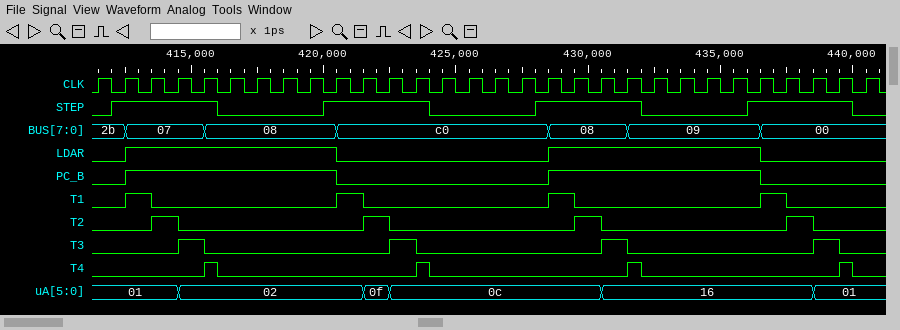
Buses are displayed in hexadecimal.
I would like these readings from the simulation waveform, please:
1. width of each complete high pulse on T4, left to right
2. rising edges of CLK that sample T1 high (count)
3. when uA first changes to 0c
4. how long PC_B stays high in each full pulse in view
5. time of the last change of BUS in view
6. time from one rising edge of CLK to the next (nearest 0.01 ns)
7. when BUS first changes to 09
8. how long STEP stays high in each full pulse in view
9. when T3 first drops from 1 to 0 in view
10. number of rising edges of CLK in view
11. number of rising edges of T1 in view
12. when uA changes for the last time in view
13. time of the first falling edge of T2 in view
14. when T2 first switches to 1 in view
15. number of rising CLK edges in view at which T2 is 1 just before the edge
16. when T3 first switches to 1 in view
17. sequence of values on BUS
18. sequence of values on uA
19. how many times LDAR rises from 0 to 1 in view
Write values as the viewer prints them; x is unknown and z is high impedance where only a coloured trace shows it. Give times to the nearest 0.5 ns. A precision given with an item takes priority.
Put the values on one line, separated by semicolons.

0.5 ns, 0.5 ns, 0.5 ns, 0.5 ns; 4; 422.5 ns; 8 ns, 8 ns; 436.5 ns; 1 ns; 431.5 ns; 4 ns, 4 ns, 4 ns, 4 ns; 415.5 ns; 30; 4; 438.5 ns; 414.5 ns; 413.5 ns; 4; 414.5 ns; 2b, 07, 08, c0, 08, 09, 00; 01, 02, 0f, 0c, 16, 01; 2
